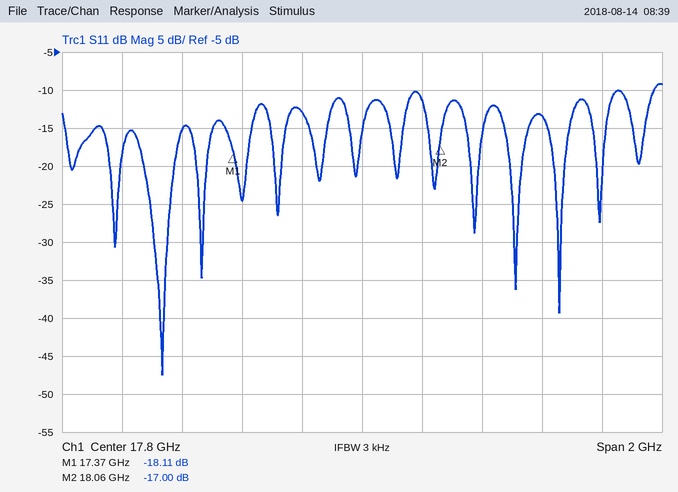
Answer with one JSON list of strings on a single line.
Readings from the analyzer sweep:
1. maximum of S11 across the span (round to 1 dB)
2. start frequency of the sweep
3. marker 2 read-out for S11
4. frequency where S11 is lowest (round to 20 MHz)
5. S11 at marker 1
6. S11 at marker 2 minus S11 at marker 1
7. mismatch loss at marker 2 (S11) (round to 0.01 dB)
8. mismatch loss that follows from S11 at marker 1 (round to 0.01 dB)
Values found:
["-9 dB", "16.8 GHz", "-17.00 dB", "17.14 GHz", "-18.11 dB", "1.11 dB", "0.09 dB", "0.07 dB"]
